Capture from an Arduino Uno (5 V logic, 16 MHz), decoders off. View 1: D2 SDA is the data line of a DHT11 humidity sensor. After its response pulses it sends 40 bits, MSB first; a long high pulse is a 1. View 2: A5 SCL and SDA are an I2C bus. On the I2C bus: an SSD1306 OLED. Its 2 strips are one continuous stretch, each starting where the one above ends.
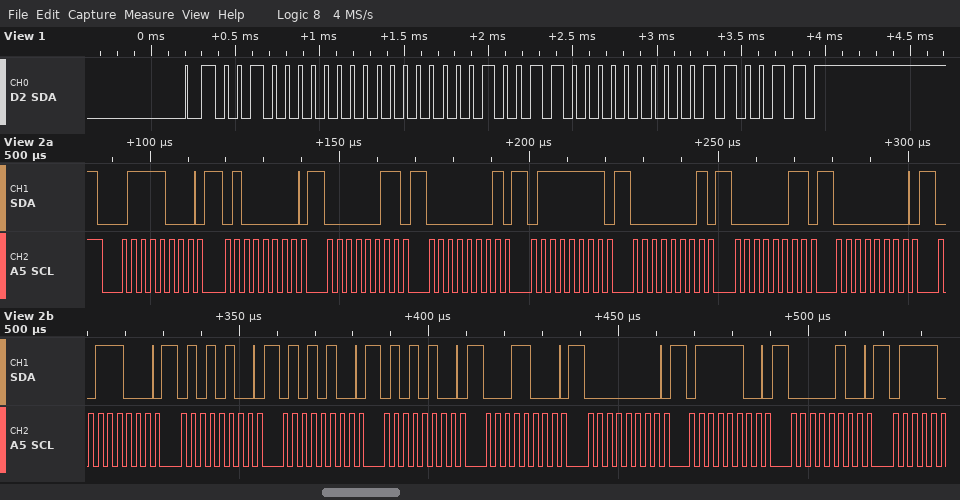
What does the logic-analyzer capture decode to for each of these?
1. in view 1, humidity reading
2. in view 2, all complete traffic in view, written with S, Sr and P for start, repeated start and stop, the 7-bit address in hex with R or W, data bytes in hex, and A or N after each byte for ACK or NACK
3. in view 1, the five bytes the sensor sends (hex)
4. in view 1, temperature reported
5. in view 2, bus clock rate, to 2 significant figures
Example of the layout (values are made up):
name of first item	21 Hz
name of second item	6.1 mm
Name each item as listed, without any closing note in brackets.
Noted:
in view 1, humidity reading	32 %
in view 2, all complete traffic in view, written with S, Sr and P for start, repeated start and stop, the 7-bit address in hex with R or W, data bytes in hex, and A or N after each byte for ACK or NACK	S 3CW A 40 A 03 A 01 A 7F A 01 A 03 A 00 A 38 A 54 A 54 A 54 A 18 A 00 A 7C A 04 A
in view 1, the five bytes the sensor sends	20 00 13 00 33
in view 1, temperature reported	19.0 °C
in view 2, bus clock rate, to 2 significant figures	400 kHz
